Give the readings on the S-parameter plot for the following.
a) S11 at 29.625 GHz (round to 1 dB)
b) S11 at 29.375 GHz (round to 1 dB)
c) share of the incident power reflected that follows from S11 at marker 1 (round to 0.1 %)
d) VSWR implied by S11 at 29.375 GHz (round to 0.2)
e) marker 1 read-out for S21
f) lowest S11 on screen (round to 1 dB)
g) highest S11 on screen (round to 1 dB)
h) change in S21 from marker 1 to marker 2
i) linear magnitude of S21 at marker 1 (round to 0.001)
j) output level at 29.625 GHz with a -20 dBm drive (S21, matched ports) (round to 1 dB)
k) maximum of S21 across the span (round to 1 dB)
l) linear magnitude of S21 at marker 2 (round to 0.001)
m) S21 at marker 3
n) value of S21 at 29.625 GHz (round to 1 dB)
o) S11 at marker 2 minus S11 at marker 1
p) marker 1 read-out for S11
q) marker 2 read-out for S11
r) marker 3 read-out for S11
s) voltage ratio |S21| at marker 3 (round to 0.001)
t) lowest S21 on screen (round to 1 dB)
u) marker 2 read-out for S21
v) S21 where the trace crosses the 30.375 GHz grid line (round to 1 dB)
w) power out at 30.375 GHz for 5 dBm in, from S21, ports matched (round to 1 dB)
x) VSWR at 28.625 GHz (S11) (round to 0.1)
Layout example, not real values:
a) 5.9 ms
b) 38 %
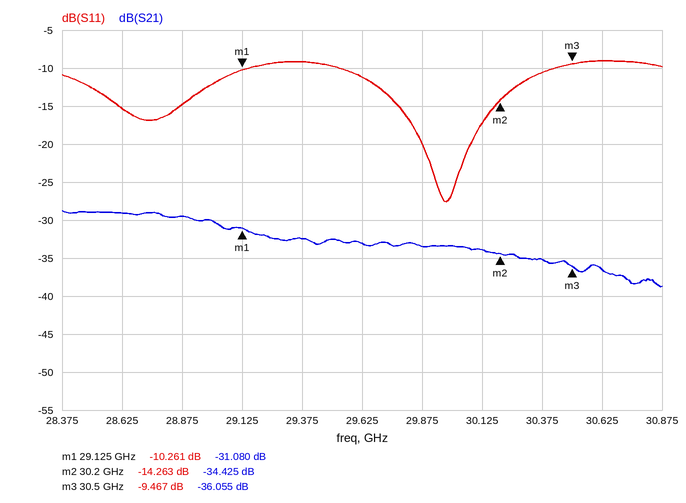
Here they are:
a) -11 dB
b) -9 dB
c) 9.4 %
d) 2.0
e) -31.080 dB
f) -28 dB
g) -9 dB
h) -3.345 dB
i) 0.028
j) -53 dBm
k) -29 dB
l) 0.019
m) -36.055 dB
n) -33 dB
o) -4.002 dB
p) -10.261 dB
q) -14.263 dB
r) -9.467 dB
s) 0.016
t) -39 dB
u) -34.425 dB
v) -35 dB
w) -30 dBm
x) 1.4
